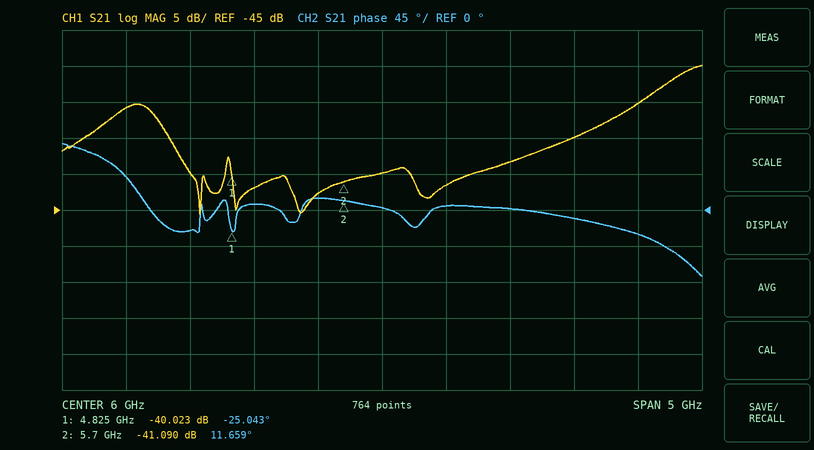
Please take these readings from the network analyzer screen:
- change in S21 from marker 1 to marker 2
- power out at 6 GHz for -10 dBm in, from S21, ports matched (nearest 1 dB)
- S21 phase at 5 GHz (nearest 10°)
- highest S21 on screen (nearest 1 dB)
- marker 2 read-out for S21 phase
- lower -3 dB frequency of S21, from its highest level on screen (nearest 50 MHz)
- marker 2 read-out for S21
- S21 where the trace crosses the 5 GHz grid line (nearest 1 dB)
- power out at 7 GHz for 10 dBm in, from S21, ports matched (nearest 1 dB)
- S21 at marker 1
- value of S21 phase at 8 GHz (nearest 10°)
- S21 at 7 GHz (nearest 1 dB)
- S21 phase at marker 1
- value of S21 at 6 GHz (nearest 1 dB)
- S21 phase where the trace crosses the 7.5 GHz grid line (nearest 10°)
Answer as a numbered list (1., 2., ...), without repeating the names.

1. -1.067 dB
2. -50 dBm
3. 10°
4. -25 dB
5. 11.659°
6. 8.20 GHz
7. -41.090 dB
8. -42 dB
9. -28 dBm
10. -40.023 dB
11. -30°
12. -38 dB
13. -25.043°
14. -40 dB
15. -10°
